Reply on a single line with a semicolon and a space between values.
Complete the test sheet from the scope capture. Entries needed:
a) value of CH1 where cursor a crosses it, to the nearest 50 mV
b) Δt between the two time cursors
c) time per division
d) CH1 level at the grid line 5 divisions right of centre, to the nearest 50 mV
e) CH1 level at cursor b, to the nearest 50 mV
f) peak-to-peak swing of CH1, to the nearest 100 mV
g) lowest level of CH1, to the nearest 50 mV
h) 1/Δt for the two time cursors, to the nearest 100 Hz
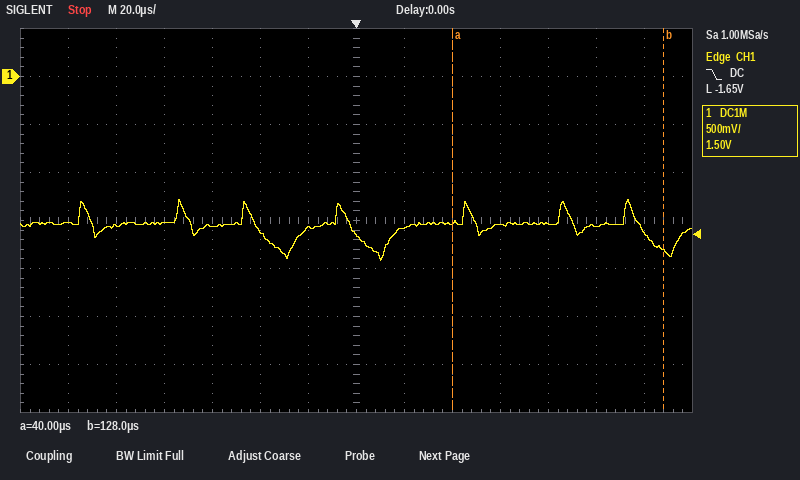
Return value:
-1.50 V; 88 µs; 20 µs; -1.55 V; -1.80 V; 600 mV; -1.90 V; 11.4 kHz
